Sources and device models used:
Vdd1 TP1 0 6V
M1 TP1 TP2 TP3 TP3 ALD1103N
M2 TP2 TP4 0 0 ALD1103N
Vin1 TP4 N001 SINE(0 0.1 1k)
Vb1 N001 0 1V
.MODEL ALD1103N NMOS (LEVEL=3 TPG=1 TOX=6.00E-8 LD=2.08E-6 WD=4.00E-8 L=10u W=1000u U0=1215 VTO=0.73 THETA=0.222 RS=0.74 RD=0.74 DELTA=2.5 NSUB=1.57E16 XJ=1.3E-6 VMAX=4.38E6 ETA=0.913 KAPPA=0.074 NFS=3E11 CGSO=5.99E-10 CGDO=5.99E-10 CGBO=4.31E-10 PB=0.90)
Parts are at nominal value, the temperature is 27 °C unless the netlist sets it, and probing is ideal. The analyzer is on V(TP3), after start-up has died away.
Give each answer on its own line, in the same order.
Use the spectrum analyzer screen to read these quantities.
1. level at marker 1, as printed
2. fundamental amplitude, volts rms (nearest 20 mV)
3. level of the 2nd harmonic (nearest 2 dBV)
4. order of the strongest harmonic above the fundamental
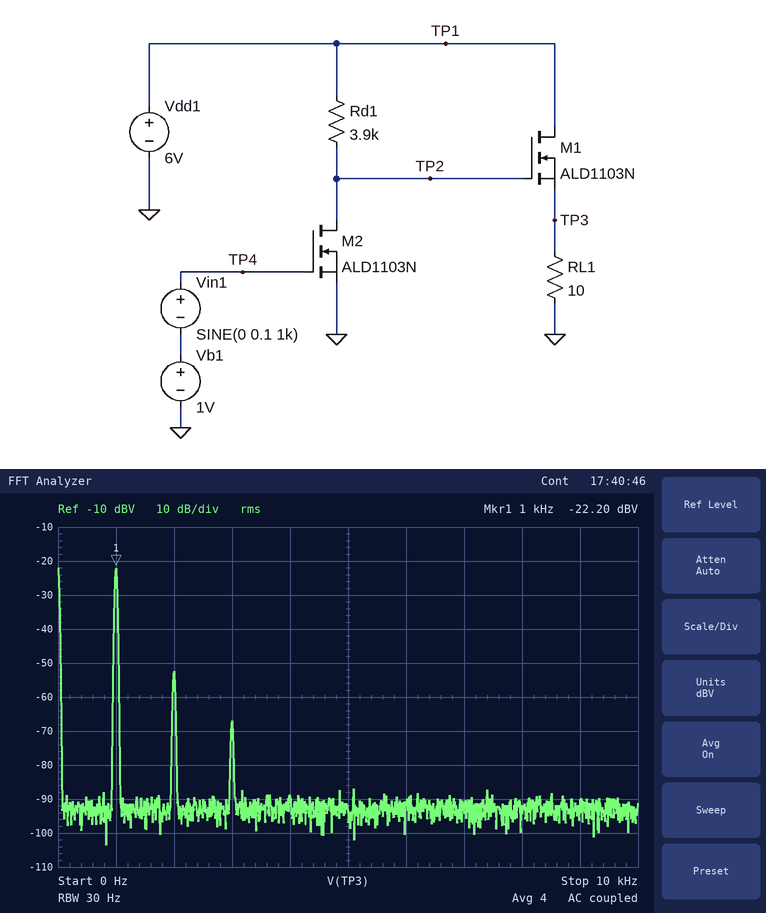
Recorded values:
-22.20 dBV
80 mV
-52 dBV
2
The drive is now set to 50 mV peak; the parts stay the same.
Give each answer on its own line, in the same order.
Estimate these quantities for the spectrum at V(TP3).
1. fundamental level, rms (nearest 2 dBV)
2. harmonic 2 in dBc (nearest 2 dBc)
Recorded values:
-28 dBV
-36 dBc
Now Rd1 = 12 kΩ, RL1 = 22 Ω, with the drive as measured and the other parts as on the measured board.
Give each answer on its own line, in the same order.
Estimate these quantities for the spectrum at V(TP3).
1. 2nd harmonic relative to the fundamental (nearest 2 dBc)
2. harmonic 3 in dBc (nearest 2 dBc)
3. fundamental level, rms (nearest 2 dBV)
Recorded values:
-6 dBc
-26 dBc
-20 dBV
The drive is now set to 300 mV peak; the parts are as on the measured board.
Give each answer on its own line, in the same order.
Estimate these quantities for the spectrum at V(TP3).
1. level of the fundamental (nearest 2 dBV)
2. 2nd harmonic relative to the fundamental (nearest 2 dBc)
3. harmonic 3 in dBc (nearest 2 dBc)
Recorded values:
-14 dBV
-28 dBc
-20 dBc
